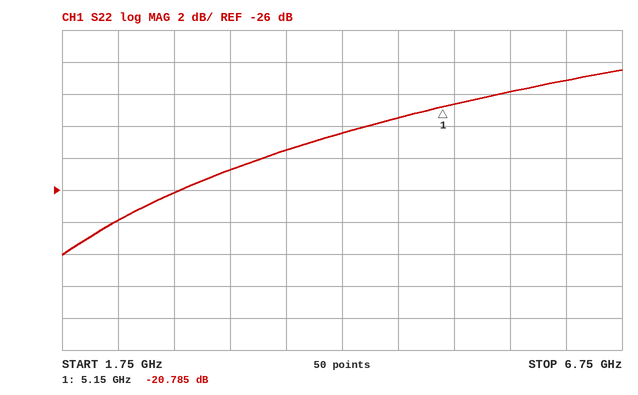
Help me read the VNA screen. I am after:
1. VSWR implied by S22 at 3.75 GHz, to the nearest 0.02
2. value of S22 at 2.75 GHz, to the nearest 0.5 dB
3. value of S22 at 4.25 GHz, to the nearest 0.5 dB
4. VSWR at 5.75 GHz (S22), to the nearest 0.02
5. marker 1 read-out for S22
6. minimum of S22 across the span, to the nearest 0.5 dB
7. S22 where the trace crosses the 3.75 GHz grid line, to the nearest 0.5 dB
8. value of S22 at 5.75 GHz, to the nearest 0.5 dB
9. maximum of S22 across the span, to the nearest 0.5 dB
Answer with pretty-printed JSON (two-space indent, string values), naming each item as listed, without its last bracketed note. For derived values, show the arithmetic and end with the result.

{
  "VSWR implied by S22 at 3.75 GHz, to the nearest 0.02": "|Γ| = 10^(-23.5/20) = 0.0668; VSWR = (1 + 0.0668)/(1 − 0.0668) ≈ 1.14",
  "value of S22 at 2.75 GHz, to the nearest 0.5 dB": "-26.0 dB",
  "value of S22 at 4.25 GHz, to the nearest 0.5 dB": "-22.5 dB",
  "VSWR at 5.75 GHz (S22), to the nearest 0.02": "|Γ| = 10^(-20/20) = 0.1000; VSWR = (1 + 0.1000)/(1 − 0.1000) ≈ 1.22",
  "marker 1 read-out for S22": "-20.785 dB",
  "minimum of S22 across the span, to the nearest 0.5 dB": "-30.0 dB",
  "S22 where the trace crosses the 3.75 GHz grid line, to the nearest 0.5 dB": "-23.5 dB",
  "value of S22 at 5.75 GHz, to the nearest 0.5 dB": "-20.0 dB",
  "maximum of S22 across the span, to the nearest 0.5 dB": "-18.5 dB"
}
